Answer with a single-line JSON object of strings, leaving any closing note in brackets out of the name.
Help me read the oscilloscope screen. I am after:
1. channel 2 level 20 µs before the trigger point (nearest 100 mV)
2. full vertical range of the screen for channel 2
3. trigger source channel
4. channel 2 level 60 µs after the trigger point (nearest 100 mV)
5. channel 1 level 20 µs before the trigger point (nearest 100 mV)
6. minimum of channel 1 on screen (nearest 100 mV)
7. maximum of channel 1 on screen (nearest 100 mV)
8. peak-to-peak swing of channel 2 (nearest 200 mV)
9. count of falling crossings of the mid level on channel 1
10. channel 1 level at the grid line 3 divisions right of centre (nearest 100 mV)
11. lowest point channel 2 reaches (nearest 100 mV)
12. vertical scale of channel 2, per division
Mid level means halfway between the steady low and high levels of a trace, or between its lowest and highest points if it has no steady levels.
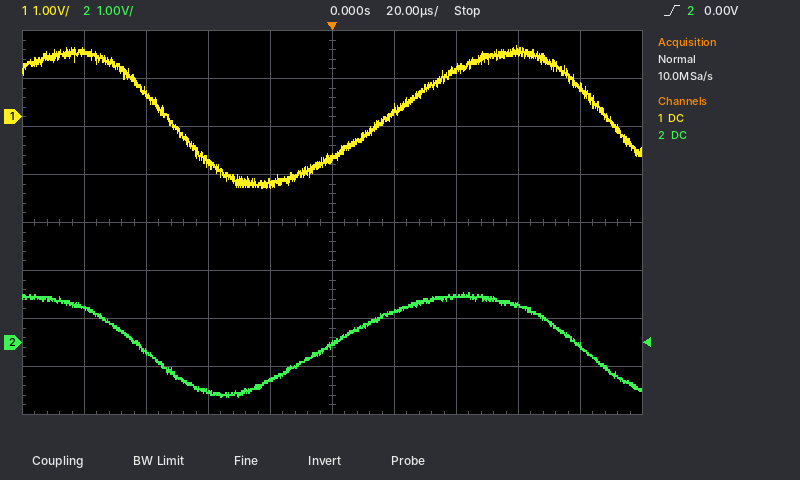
{"channel 2 level 20 µs before the trigger point": "-800 mV", "full vertical range of the screen for channel 2": "8 V", "trigger source channel": "channel 2", "channel 2 level 60 µs after the trigger point": "800 mV", "channel 1 level 20 µs before the trigger point": "-1.4 V", "minimum of channel 1 on screen": "-1.5 V", "maximum of channel 1 on screen": "1.5 V", "peak-to-peak swing of channel 2": "2.2 V", "count of falling crossings of the mid level on channel 1": "2", "channel 1 level at the grid line 3 divisions right of centre": "1.4 V", "lowest point channel 2 reaches": "-1.1 V", "vertical scale of channel 2, per division": "1 V"}
